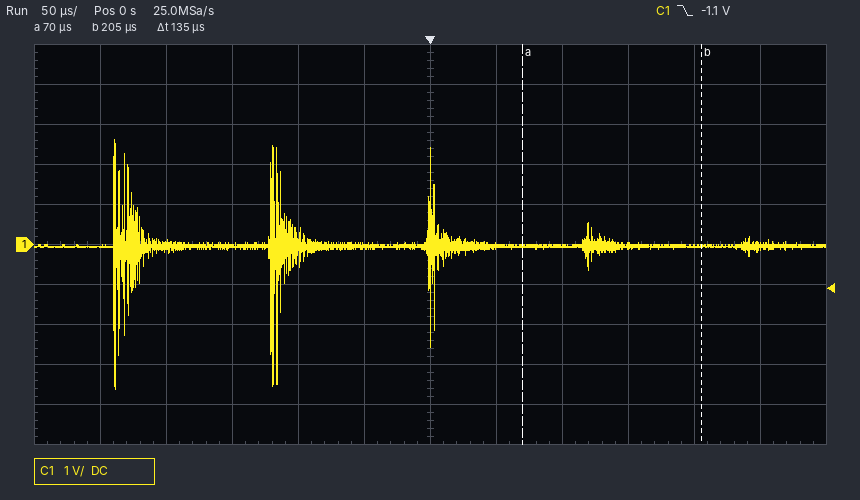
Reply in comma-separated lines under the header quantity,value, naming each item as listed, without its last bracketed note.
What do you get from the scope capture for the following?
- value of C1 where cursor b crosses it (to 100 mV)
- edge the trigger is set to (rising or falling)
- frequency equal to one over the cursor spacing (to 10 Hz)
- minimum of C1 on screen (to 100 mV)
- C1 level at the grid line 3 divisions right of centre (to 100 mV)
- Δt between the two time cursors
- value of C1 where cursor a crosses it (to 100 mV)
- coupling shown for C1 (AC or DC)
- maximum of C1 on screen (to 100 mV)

quantity,value
value of C1 where cursor b crosses it,0.0 V
edge the trigger is set to,falling
frequency equal to one over the cursor spacing,7.41 kHz
minimum of C1 on screen,-3.6 V
C1 level at the grid line 3 divisions right of centre,0.0 V
Δt between the two time cursors,135 µs
value of C1 where cursor a crosses it,0.0 V
coupling shown for C1,DC
maximum of C1 on screen,2.6 V
